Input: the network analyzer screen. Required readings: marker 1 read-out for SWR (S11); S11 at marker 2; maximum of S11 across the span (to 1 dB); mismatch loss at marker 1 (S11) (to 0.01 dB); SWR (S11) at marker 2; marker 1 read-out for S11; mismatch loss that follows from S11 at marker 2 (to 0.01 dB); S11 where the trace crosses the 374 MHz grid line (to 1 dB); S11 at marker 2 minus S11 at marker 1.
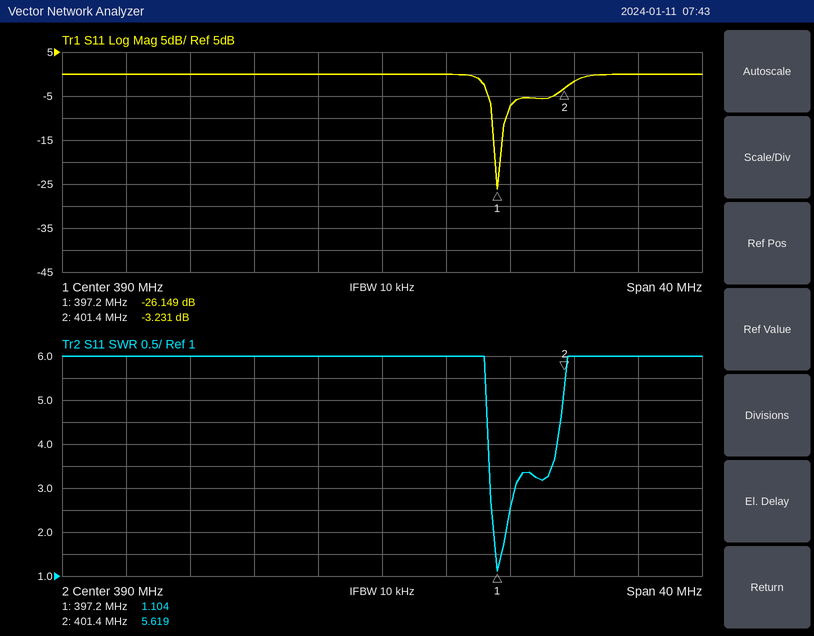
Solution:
1.104
-3.231 dB
0 dB
0.01 dB
5.619
-26.149 dB
2.80 dB
0 dB
22.918 dB
